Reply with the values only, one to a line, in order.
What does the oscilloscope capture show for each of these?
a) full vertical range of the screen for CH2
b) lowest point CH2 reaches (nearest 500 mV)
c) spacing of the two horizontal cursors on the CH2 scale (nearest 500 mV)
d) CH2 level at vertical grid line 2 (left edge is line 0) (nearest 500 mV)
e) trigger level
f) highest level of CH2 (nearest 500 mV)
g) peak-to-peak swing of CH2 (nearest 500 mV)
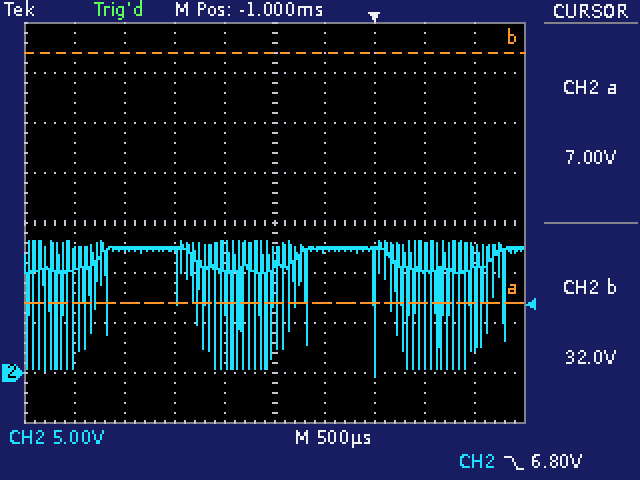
40 V
-500 mV
25.0 V
12.5 V
6.80 V
13.0 V
13.5 V
